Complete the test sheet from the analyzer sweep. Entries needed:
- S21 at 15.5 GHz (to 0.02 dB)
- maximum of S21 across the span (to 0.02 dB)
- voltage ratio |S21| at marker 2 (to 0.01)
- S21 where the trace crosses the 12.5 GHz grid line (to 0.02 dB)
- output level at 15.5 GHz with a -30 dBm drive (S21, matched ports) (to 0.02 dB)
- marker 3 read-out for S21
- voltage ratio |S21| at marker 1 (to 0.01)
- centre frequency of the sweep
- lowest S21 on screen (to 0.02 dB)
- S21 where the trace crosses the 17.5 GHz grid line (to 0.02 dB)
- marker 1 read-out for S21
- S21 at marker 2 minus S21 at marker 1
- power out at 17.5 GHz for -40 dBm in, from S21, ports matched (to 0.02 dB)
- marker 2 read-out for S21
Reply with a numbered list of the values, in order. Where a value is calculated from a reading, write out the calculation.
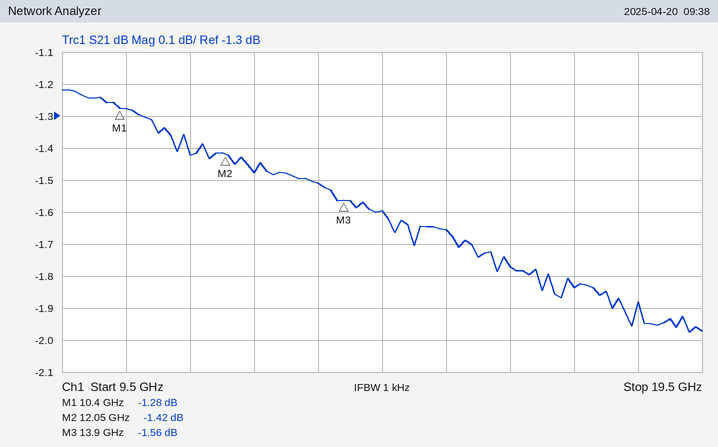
1. -1.66 dB
2. -1.22 dB
3. 10^(-1.42/20) ≈ 0.85
4. -1.48 dB
5. -30 dBm + (-1.66 dB) = -31.66 dBm
6. -1.56 dB
7. 10^(-1.28/20) ≈ 0.86
8. 14.5 GHz
9. -1.98 dB
10. -1.84 dB
11. -1.28 dB
12. -1.42 − (-1.28) = -0.14 dB
13. -40 dBm + (-1.84 dB) = -41.84 dBm
14. -1.42 dB
